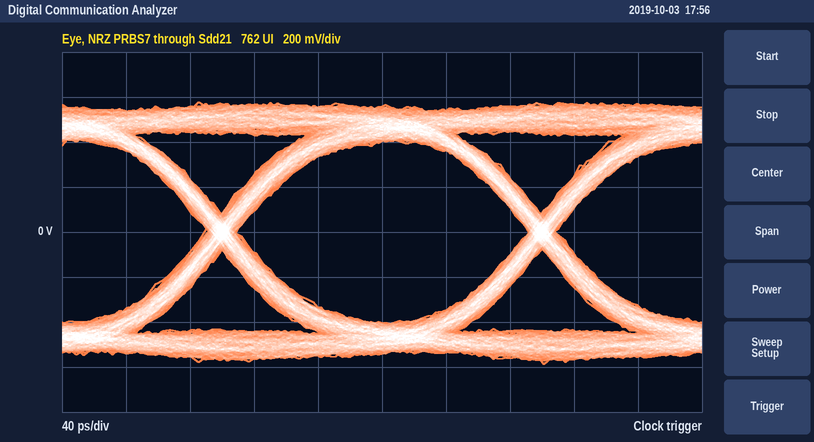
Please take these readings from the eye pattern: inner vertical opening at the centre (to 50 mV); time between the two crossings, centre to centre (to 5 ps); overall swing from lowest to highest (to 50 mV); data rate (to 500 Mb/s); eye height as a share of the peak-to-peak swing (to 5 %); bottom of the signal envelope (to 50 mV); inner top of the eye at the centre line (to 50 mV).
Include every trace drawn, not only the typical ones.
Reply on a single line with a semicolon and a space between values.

800 mV; 200 ps; 1.15 V; 5.0 Gb/s; 70 %; -600 mV; 400 mV
